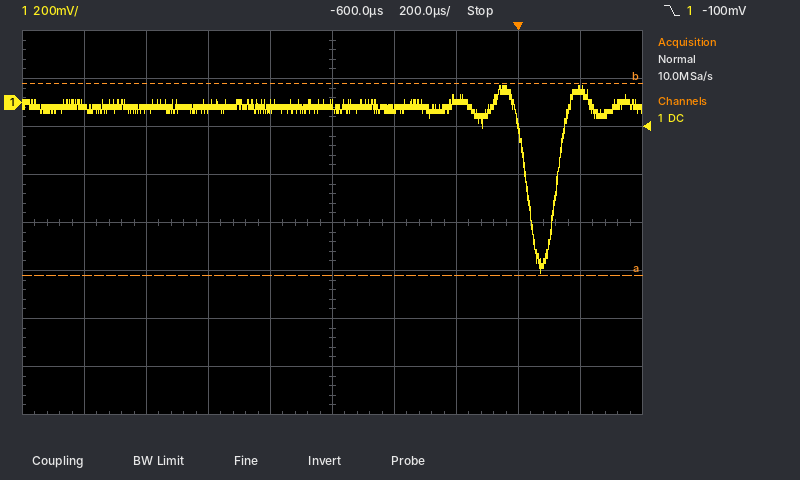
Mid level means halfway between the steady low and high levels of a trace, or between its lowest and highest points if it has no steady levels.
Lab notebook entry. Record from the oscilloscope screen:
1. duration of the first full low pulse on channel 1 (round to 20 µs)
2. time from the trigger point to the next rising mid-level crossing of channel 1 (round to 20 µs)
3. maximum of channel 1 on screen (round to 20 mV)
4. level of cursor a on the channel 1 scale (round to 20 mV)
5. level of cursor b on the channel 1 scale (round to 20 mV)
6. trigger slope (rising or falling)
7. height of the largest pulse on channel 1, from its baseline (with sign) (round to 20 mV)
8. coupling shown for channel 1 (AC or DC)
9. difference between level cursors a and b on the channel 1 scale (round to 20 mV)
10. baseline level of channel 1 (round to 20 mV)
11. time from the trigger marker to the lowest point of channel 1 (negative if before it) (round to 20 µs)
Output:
100 µs
120 µs
80 mV
-720 mV
80 mV
falling
-700 mV
DC
800 mV
-20 mV
+80 µs
